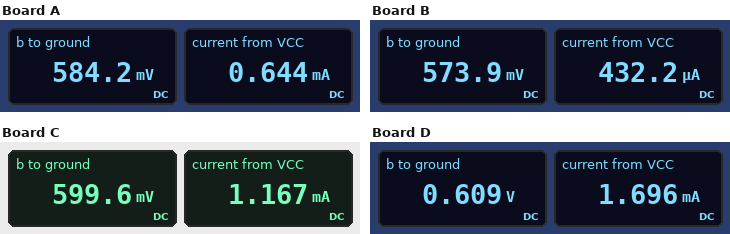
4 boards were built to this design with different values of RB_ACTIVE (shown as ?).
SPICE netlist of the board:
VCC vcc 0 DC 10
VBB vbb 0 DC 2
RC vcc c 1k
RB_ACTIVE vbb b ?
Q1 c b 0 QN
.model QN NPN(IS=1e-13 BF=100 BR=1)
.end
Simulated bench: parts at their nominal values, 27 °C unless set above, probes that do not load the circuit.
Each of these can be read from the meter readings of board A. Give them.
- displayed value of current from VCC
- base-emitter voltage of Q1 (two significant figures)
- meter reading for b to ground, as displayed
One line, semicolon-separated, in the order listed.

0.644 mA; 580 mV; 584.2 mV
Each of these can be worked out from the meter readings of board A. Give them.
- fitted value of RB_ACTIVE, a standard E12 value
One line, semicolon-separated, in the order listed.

220 kΩ
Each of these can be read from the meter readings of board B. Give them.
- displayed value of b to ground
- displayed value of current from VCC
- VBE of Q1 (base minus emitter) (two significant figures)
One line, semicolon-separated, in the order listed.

573.9 mV; 432.2 µA; 570 mV
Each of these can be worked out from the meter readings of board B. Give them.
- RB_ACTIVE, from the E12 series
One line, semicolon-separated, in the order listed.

330 kΩ
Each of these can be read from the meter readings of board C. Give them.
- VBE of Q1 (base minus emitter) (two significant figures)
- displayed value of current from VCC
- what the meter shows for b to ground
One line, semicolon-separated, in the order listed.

600 mV; 1.167 mA; 599.6 mV
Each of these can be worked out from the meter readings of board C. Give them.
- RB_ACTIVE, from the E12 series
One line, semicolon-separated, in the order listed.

120 kΩ
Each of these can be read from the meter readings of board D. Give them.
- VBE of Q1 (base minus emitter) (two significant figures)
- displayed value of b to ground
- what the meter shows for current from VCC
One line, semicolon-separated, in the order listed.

610 mV; 0.609 V; 1.696 mA
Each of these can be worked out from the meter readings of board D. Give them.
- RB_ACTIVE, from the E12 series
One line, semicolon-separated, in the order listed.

82 kΩ
